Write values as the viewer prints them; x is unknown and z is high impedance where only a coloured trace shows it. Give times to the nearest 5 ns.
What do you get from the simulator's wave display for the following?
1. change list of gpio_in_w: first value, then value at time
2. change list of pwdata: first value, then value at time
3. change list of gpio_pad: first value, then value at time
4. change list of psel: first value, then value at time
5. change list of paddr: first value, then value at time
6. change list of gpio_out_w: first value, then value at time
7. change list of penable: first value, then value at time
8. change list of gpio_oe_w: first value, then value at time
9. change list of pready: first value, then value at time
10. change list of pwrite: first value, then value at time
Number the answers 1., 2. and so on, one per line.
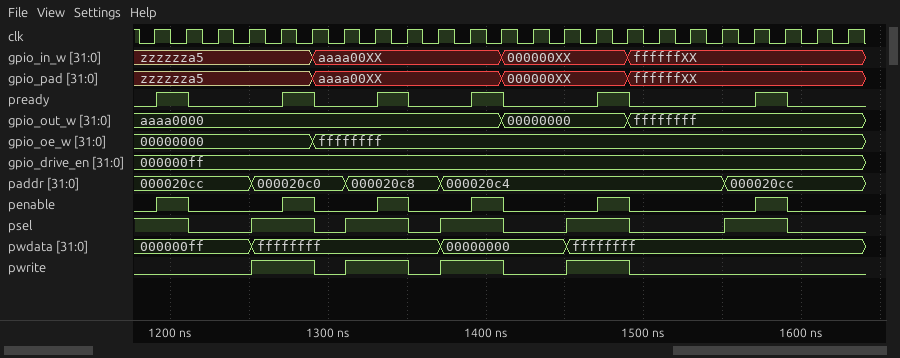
1. zzzzzza5, aaaa00XX at 1290 ns, 000000XX at 1410 ns, ffffffXX at 1490 ns
2. 000000ff, ffffffff at 1250 ns, 00000000 at 1370 ns, ffffffff at 1450 ns
3. zzzzzza5, aaaa00XX at 1290 ns, 000000XX at 1410 ns, ffffffXX at 1490 ns
4. 1, 0 at 1210 ns, 1 at 1250 ns, 0 at 1290 ns, 1 at 1310 ns, 0 at 1350 ns, 1 at 1370 ns, 0 at 1410 ns, 1 at 1450 ns, 0 at 1490 ns, 1 at 1550 ns, 0 at 1590 ns
5. 000020cc, 000020c0 at 1250 ns, 000020c8 at 1310 ns, 000020c4 at 1370 ns, 000020cc at 1550 ns
6. aaaa0000, 00000000 at 1410 ns, ffffffff at 1490 ns
7. 0, 1 at 1190 ns, 0 at 1210 ns, 1 at 1270 ns, 0 at 1290 ns, 1 at 1330 ns, 0 at 1350 ns, 1 at 1390 ns, 0 at 1410 ns, 1 at 1470 ns, 0 at 1490 ns, 1 at 1570 ns, 0 at 1590 ns
8. 00000000, ffffffff at 1290 ns
9. 0, 1 at 1190 ns, 0 at 1210 ns, 1 at 1270 ns, 0 at 1290 ns, 1 at 1330 ns, 0 at 1350 ns, 1 at 1390 ns, 0 at 1410 ns, 1 at 1470 ns, 0 at 1490 ns, 1 at 1570 ns, 0 at 1590 ns
10. 0, 1 at 1250 ns, 0 at 1290 ns, 1 at 1310 ns, 0 at 1350 ns, 1 at 1370 ns, 0 at 1410 ns, 1 at 1450 ns, 0 at 1490 ns
